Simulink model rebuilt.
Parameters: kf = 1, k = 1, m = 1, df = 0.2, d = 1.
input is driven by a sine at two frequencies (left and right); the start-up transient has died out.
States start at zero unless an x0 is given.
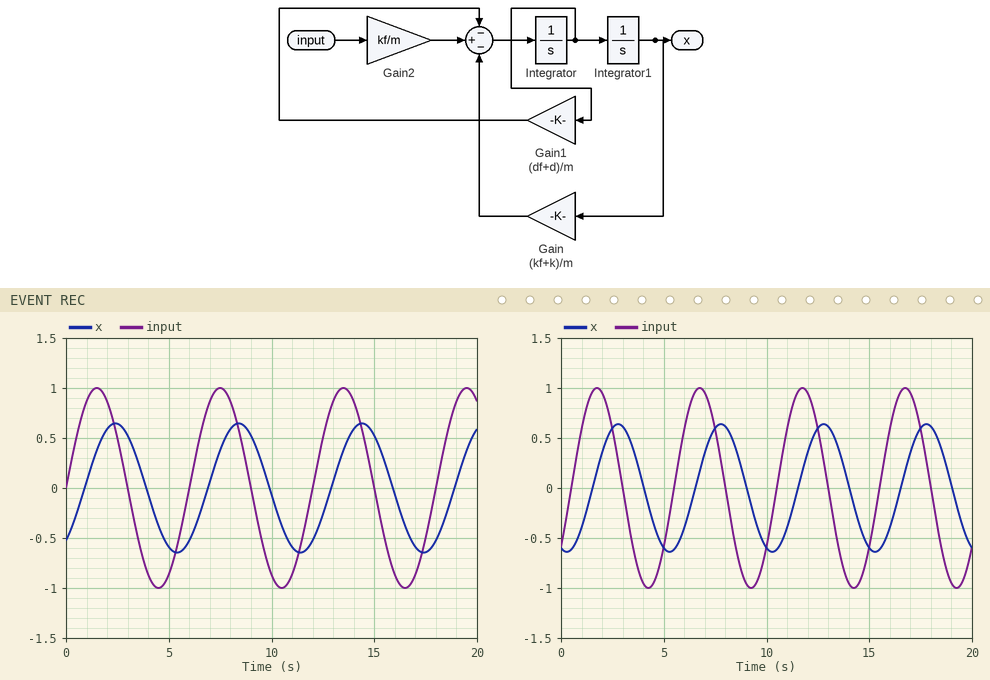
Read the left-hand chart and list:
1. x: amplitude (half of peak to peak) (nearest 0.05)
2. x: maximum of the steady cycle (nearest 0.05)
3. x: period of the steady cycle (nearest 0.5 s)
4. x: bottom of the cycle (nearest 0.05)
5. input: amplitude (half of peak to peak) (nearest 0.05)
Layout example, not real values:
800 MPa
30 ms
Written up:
0.65
0.65
6.0 s
-0.65
1.00
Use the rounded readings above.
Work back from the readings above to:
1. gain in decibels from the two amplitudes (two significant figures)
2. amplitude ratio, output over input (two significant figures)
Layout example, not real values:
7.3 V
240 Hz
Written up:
-3.7 dB
0.65
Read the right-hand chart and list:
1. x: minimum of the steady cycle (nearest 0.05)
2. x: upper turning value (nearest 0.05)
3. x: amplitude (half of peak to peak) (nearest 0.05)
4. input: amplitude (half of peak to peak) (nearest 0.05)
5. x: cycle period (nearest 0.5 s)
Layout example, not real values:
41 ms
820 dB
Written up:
-0.65
0.65
0.65
1.00
5.0 s
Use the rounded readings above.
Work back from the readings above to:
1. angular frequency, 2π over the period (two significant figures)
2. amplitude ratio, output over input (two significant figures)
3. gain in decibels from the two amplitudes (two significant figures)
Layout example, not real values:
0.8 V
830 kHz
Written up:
1.3 rad/s
0.65
-3.7 dB
